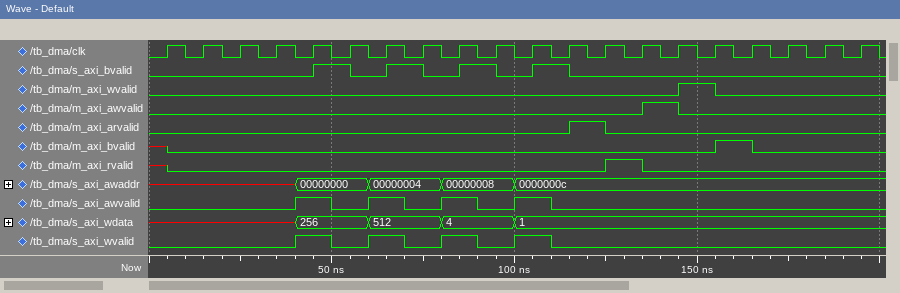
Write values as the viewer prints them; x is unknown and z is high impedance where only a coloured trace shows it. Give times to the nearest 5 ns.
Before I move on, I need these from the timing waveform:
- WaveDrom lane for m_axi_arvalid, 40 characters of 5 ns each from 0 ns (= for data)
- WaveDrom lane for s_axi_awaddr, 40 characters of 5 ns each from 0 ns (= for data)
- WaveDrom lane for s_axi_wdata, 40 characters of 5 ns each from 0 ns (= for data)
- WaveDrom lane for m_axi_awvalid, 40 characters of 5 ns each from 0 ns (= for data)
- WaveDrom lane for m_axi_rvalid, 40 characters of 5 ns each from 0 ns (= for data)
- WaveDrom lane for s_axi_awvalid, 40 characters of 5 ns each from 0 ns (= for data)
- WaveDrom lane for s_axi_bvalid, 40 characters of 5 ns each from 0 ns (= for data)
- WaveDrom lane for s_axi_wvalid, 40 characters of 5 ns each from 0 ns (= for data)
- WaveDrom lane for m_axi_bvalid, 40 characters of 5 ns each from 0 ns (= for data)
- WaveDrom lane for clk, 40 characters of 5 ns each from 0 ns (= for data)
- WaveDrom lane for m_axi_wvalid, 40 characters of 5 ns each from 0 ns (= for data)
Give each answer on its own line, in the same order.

{name: 'm_axi_arvalid', wave: '0......................1.0..............'}
{name: 's_axi_awaddr', wave: 'x.......=...=...=...=...................', data: '00000000 00000004 00000008 0000000c'}
{name: 's_axi_wdata', wave: 'x.......=...=...=...=...................', data: '256 512 4 1'}
{name: 'm_axi_awvalid', wave: '0..........................1.0..........'}
{name: 'm_axi_rvalid', wave: 'x0.......................1.0............'}
{name: 's_axi_awvalid', wave: '0.......1.0.1.0.1.0.1.0.................'}
{name: 's_axi_bvalid', wave: '0........1.0.1.0.1.0.1.0................'}
{name: 's_axi_wvalid', wave: '0.......1.0.1.0.1.0.1.0.................'}
{name: 'm_axi_bvalid', wave: 'x0.............................1.0......'}
{name: 'clk', wave: '0101010101010101010101010101010101010101'}
{name: 'm_axi_wvalid', wave: '0............................1.0........'}
